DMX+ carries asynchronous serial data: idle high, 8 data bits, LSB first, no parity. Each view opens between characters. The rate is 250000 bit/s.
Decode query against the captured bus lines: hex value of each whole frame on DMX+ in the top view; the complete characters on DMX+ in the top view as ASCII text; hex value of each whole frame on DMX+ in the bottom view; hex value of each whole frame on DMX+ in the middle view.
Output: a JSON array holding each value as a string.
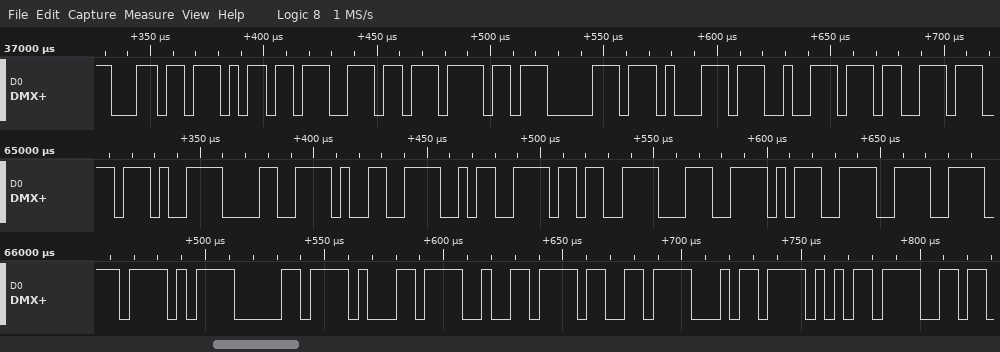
["6C, 6D, 6E, 6F, 70, 71, 72, 73", "\"lmnopqrs\"", "AF, B0, B1, B2, B3, B4, B5", "97, 98, 99, 9A, 9B, 9C, 9D, 9E"]
